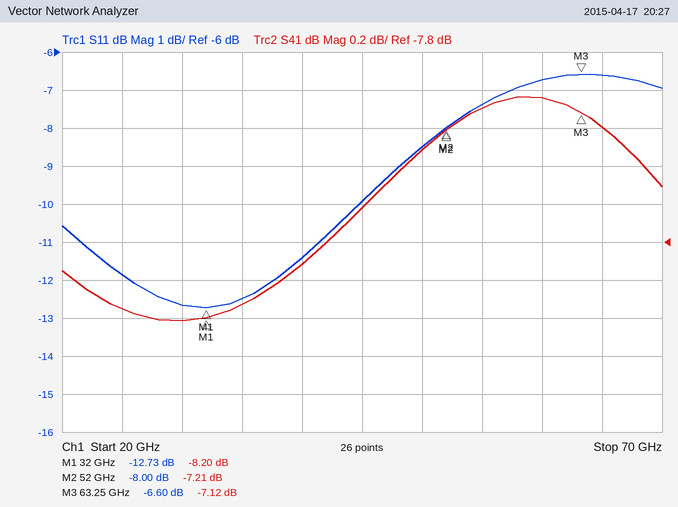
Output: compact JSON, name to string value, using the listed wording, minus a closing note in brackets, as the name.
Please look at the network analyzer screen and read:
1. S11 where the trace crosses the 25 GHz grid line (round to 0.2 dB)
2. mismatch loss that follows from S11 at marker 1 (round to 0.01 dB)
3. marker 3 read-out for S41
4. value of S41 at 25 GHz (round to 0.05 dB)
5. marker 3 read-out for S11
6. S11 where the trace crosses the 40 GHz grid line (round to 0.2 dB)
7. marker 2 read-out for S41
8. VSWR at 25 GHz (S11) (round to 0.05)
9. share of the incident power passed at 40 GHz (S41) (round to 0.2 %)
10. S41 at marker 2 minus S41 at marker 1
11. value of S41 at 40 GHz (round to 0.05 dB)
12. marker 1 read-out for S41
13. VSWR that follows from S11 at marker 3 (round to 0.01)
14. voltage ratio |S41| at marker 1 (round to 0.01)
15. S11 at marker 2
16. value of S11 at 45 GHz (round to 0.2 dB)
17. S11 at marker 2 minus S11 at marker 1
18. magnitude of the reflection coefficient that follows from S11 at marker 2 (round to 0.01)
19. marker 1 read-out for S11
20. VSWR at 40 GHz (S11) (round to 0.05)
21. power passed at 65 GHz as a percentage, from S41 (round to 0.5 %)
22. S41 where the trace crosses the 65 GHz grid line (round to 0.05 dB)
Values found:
{"S11 where the trace crosses the 25 GHz grid line": "-11.8 dB", "mismatch loss that follows from S11 at marker 1": "0.24 dB", "marker 3 read-out for S41": "-7.12 dB", "value of S41 at 25 GHz": "-8.15 dB", "marker 3 read-out for S11": "-6.60 dB", "S11 where the trace crosses the 40 GHz grid line": "-11.4 dB", "marker 2 read-out for S41": "-7.21 dB", "VSWR at 25 GHz (S11)": "1.70", "share of the incident power passed at 40 GHz (S41)": "16.2 %", "S41 at marker 2 minus S41 at marker 1": "0.99 dB", "value of S41 at 40 GHz": "-7.90 dB", "marker 1 read-out for S41": "-8.20 dB", "VSWR that follows from S11 at marker 3": "2.76", "voltage ratio |S41| at marker 1": "0.39", "S11 at marker 2": "-8.00 dB", "value of S11 at 45 GHz": "-10.0 dB", "S11 at marker 2 minus S11 at marker 1": "4.73 dB", "magnitude of the reflection coefficient that follows from S11 at marker 2": "0.40", "marker 1 read-out for S11": "-12.73 dB", "VSWR at 40 GHz (S11)": "1.75", "power passed at 65 GHz as a percentage, from S41": "19.0 %", "S41 where the trace crosses the 65 GHz grid line": "-7.20 dB"}
